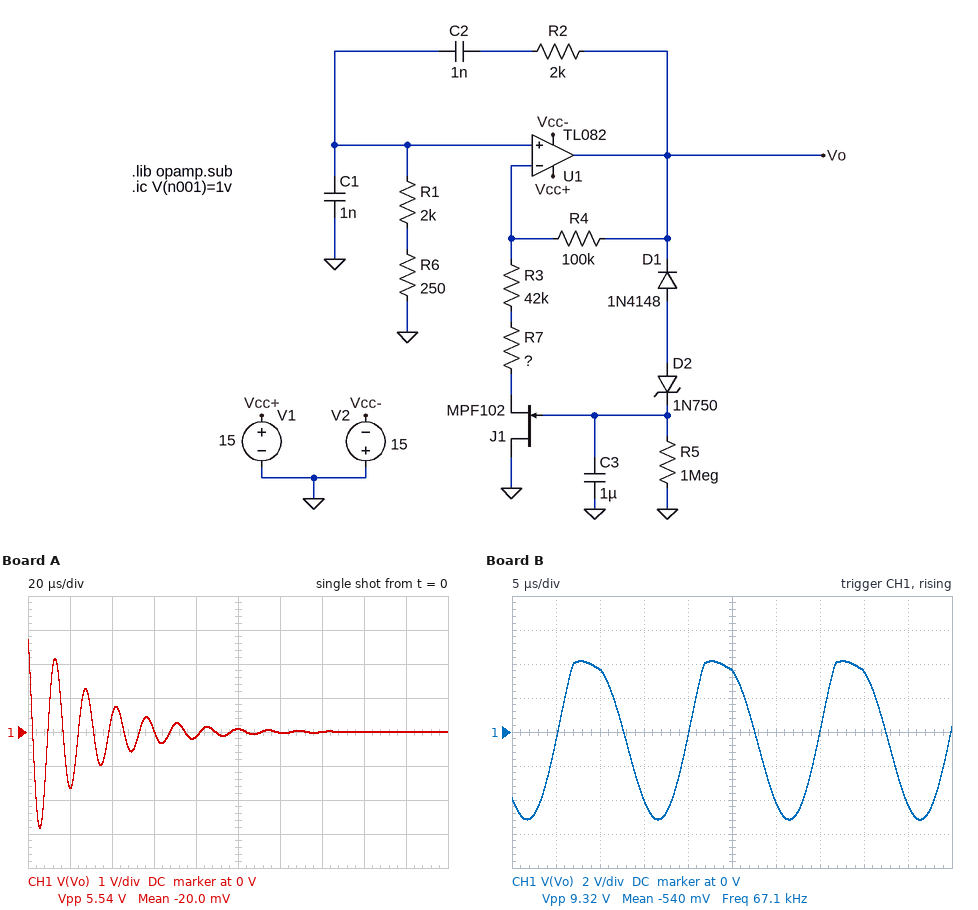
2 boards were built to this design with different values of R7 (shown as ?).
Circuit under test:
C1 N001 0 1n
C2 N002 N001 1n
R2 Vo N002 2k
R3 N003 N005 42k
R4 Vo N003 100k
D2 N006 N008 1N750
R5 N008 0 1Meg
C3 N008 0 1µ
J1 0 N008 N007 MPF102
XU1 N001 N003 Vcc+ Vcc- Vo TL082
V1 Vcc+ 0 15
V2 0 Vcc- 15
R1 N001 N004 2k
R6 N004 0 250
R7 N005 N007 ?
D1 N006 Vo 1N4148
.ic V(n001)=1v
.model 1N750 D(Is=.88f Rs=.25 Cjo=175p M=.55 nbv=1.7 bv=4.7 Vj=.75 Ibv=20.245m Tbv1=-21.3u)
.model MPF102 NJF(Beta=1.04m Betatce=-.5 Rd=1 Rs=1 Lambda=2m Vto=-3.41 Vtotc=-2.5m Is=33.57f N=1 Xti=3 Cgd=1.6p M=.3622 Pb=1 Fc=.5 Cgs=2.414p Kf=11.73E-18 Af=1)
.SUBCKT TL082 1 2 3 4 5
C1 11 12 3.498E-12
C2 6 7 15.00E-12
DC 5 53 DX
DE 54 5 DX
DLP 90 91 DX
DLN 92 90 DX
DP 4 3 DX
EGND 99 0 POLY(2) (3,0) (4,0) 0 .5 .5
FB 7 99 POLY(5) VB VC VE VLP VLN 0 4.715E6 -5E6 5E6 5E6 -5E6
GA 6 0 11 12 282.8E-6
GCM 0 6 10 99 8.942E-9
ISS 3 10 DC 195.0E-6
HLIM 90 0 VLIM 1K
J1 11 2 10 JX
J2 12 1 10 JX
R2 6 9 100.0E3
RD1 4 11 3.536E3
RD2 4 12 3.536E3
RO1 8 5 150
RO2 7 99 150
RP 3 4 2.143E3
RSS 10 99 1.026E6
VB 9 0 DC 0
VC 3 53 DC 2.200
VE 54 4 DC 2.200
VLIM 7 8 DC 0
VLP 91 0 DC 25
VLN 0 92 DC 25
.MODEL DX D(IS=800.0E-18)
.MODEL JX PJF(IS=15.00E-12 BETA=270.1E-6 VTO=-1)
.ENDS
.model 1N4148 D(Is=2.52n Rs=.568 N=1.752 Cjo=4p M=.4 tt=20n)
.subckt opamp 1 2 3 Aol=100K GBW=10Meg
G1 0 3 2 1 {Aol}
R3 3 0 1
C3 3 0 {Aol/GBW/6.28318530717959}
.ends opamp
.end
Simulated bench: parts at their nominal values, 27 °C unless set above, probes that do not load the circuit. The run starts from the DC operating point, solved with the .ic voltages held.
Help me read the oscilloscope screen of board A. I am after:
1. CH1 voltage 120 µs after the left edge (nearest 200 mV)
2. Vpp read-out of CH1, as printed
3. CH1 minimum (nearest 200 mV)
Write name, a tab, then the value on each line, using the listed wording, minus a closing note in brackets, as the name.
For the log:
CH1 voltage 120 µs after the left edge	0 V
Vpp read-out of CH1, as printed	5.54 V
CH1 minimum	-2.8 V
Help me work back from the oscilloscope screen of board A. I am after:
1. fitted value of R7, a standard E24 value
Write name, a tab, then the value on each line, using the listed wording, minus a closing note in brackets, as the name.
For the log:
fitted value of R7, a standard E24 value	16 kΩ
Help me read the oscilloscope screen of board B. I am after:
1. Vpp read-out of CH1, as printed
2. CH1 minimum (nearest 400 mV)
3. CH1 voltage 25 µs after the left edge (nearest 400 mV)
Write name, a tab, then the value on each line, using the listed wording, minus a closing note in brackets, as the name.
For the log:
Vpp read-out of CH1, as printed	9.32 V
CH1 minimum	-5.2 V
CH1 voltage 25 µs after the left edge	3.6 V
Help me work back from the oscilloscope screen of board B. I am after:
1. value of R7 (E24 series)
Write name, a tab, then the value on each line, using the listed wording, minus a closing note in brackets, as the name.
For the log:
value of R7	3.6 kΩ
